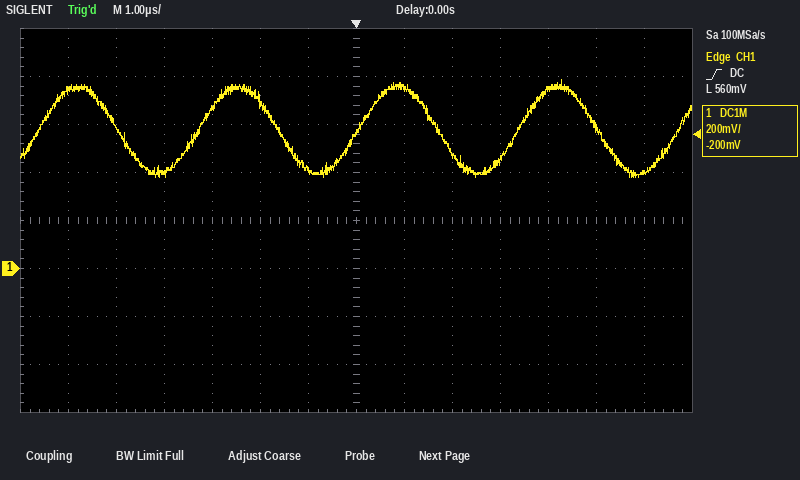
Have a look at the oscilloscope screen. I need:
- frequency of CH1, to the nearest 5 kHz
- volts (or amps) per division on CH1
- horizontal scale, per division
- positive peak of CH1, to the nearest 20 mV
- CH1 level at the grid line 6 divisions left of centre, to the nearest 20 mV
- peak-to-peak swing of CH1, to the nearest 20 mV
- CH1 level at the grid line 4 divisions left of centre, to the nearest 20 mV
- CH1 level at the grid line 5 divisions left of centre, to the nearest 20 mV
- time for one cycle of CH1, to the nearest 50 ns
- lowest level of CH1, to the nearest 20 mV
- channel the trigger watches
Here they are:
300 kHz
200 mV
1 µs
780 mV
740 mV
400 mV
400 mV
580 mV
3.35 µs
380 mV
CH1
